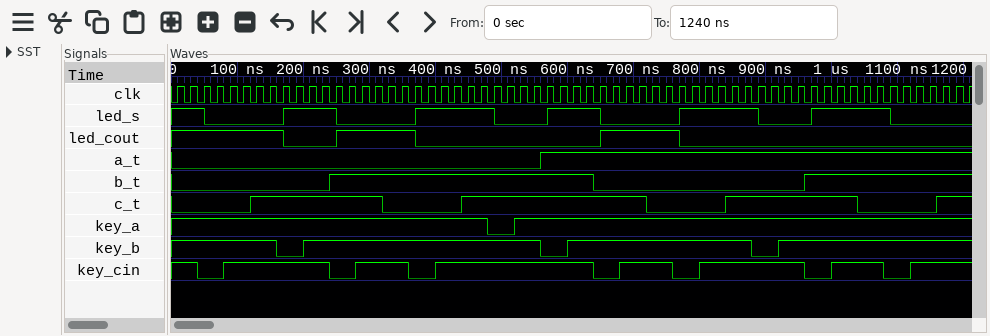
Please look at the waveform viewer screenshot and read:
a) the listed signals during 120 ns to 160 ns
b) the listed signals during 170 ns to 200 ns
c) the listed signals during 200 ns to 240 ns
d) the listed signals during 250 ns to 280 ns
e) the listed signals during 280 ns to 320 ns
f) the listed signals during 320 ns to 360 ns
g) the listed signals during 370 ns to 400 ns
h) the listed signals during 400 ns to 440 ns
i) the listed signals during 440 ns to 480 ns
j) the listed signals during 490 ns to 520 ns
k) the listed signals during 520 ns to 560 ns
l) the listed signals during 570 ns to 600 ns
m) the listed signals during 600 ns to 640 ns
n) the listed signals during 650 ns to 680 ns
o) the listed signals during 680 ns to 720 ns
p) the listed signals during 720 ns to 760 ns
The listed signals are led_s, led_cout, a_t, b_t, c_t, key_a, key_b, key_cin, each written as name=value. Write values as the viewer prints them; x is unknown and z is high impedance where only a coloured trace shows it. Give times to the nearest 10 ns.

led_s=0, led_cout=1, a_t=0, b_t=0, c_t=1, key_a=1, key_b=1, key_cin=1
led_s=1, led_cout=0, a_t=0, b_t=0, c_t=1, key_a=1, key_b=0, key_cin=1
led_s=1, led_cout=0, a_t=0, b_t=0, c_t=1, key_a=1, key_b=1, key_cin=1
led_s=0, led_cout=1, a_t=0, b_t=1, c_t=1, key_a=1, key_b=1, key_cin=0
led_s=0, led_cout=1, a_t=0, b_t=1, c_t=1, key_a=1, key_b=1, key_cin=1
led_s=0, led_cout=1, a_t=0, b_t=1, c_t=0, key_a=1, key_b=1, key_cin=1
led_s=1, led_cout=0, a_t=0, b_t=1, c_t=0, key_a=1, key_b=1, key_cin=0
led_s=1, led_cout=0, a_t=0, b_t=1, c_t=0, key_a=1, key_b=1, key_cin=1
led_s=1, led_cout=0, a_t=0, b_t=1, c_t=1, key_a=1, key_b=1, key_cin=1
led_s=0, led_cout=0, a_t=0, b_t=1, c_t=1, key_a=0, key_b=1, key_cin=1
led_s=0, led_cout=0, a_t=0, b_t=1, c_t=1, key_a=1, key_b=1, key_cin=1
led_s=1, led_cout=0, a_t=1, b_t=1, c_t=1, key_a=1, key_b=0, key_cin=1
led_s=1, led_cout=0, a_t=1, b_t=1, c_t=1, key_a=1, key_b=1, key_cin=1
led_s=0, led_cout=1, a_t=1, b_t=0, c_t=1, key_a=1, key_b=1, key_cin=0
led_s=0, led_cout=1, a_t=1, b_t=0, c_t=1, key_a=1, key_b=1, key_cin=1
led_s=0, led_cout=1, a_t=1, b_t=0, c_t=0, key_a=1, key_b=1, key_cin=1
